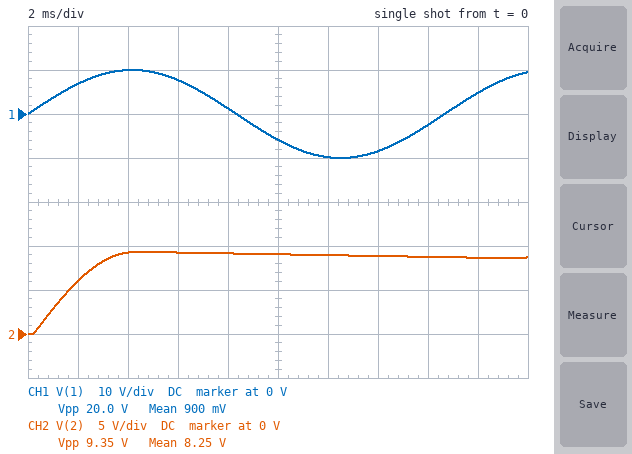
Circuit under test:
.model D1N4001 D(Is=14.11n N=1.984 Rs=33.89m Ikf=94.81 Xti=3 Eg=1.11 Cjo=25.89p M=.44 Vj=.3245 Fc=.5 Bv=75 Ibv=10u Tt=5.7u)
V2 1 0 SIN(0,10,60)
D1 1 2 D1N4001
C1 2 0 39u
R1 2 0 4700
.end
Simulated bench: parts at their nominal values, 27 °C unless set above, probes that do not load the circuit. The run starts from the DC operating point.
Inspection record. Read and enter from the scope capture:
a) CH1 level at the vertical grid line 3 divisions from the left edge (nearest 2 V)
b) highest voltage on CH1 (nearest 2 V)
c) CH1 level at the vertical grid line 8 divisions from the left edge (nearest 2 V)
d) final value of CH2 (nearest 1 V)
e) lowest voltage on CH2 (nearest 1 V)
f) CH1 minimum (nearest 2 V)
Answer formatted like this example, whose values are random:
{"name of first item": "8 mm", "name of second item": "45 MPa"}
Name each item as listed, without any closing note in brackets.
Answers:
{"CH1 level at the vertical grid line 3 divisions from the left edge": "8 V", "highest voltage on CH1": "10 V", "CH1 level at the vertical grid line 8 divisions from the left edge": "-2 V", "final value of CH2": "9 V", "lowest voltage on CH2": "0 V", "CH1 minimum": "-10 V"}
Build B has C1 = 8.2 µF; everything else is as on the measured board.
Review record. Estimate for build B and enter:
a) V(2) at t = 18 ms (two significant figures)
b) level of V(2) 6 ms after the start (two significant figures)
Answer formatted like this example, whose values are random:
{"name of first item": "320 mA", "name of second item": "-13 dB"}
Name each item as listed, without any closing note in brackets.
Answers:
{"V(2) at t = 18 ms": "6.6 V", "level of V(2) 6 ms after the start": "9.0 V"}
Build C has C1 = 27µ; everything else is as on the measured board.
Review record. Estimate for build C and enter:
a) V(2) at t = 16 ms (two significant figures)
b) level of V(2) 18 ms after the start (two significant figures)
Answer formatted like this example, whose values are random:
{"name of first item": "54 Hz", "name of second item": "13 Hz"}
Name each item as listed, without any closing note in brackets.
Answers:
{"V(2) at t = 16 ms": "8.5 V", "level of V(2) 18 ms after the start": "8.4 V"}
